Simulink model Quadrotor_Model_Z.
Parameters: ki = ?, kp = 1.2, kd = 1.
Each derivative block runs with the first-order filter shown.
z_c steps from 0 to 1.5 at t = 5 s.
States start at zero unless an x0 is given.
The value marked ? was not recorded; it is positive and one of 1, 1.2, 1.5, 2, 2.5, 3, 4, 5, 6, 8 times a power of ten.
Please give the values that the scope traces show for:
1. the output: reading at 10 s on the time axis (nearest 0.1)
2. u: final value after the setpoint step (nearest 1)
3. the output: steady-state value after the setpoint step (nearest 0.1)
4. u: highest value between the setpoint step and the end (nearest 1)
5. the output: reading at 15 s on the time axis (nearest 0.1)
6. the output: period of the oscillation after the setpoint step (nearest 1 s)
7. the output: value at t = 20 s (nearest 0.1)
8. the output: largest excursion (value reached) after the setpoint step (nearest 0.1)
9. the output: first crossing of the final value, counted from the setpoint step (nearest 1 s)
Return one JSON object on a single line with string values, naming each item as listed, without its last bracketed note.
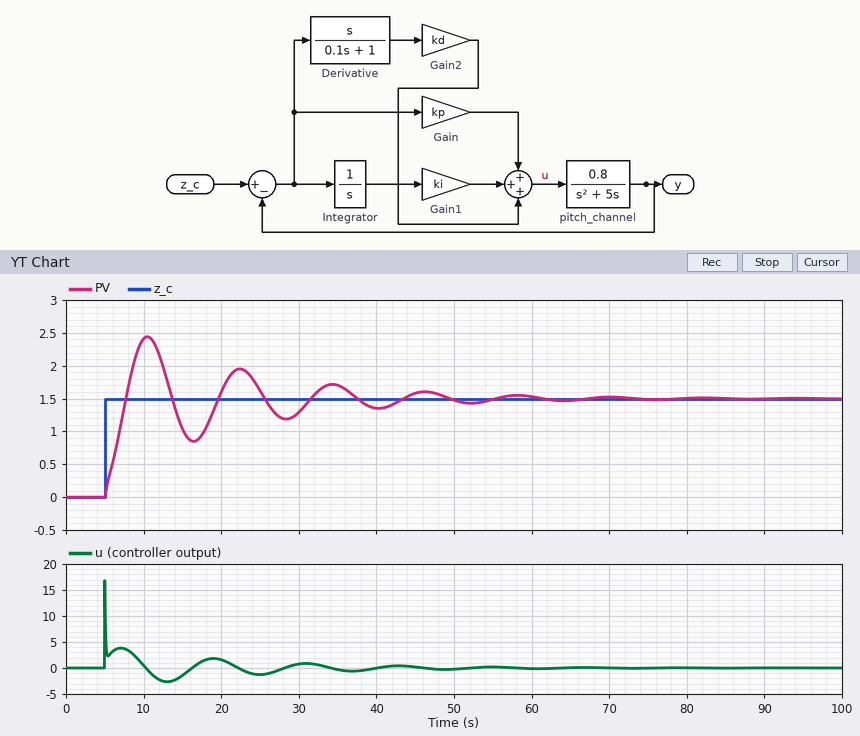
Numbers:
{"the output: reading at 10 s on the time axis": "2.4", "u: final value after the setpoint step": "0", "the output: steady-state value after the setpoint step": "1.5", "u: highest value between the setpoint step and the end": "17", "the output: reading at 15 s on the time axis": "1.0", "the output: period of the oscillation after the setpoint step": "12 s", "the output: value at t = 20 s": "1.6", "the output: largest excursion (value reached) after the setpoint step": "2.4", "the output: first crossing of the final value, counted from the setpoint step": "3 s"}
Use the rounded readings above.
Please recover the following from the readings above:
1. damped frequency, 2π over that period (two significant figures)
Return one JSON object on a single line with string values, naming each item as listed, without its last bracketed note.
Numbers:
{"damped frequency, 2π over that period": "0.52 rad/s"}
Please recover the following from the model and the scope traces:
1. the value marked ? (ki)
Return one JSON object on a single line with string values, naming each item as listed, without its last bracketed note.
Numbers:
{"the value marked ?": "2"}
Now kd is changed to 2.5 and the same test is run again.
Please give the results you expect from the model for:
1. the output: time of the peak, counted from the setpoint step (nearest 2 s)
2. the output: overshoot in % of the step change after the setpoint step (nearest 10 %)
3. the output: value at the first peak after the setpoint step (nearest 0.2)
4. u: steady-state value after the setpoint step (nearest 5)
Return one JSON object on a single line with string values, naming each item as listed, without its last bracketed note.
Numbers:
{"the output: time of the peak, counted from the setpoint step": "6 s", "the output: overshoot in % of the step change after the setpoint step": "50 %", "the output: value at the first peak after the setpoint step": "2.2", "u: steady-state value after the setpoint step": "0"}
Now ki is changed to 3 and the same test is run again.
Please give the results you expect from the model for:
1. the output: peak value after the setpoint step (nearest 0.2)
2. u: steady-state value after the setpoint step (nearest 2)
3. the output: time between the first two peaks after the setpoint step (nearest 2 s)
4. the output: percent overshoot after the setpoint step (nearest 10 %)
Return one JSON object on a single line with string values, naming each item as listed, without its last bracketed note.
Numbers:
{"the output: peak value after the setpoint step": "2.6", "u: steady-state value after the setpoint step": "0", "the output: time between the first two peaks after the setpoint step": "10 s", "the output: percent overshoot after the setpoint step": "70 %"}
